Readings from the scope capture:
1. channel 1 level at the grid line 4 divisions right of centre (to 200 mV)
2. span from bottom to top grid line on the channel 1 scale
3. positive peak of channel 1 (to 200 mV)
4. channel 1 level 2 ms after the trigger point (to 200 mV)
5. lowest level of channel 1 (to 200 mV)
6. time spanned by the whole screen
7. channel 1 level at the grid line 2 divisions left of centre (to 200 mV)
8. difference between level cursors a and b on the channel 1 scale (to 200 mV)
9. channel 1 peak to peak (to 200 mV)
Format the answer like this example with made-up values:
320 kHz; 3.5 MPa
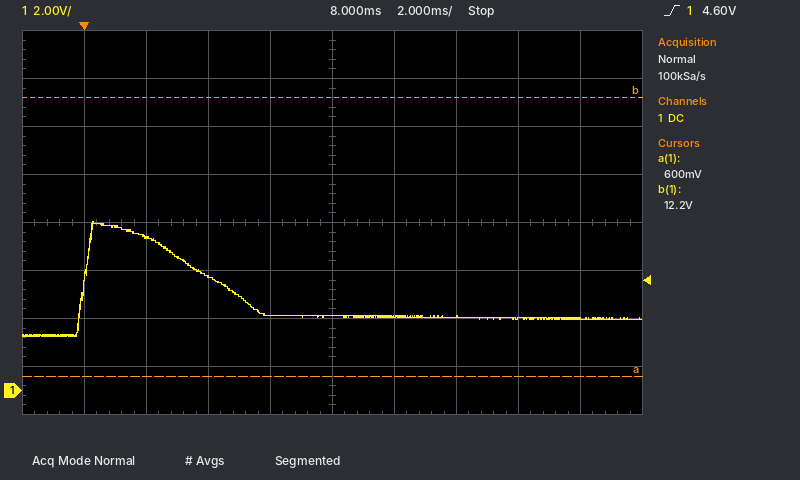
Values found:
3.0 V; 16 V; 7.0 V; 6.4 V; 2.2 V; 20 ms; 4.8 V; 11.6 V; 4.8 V
